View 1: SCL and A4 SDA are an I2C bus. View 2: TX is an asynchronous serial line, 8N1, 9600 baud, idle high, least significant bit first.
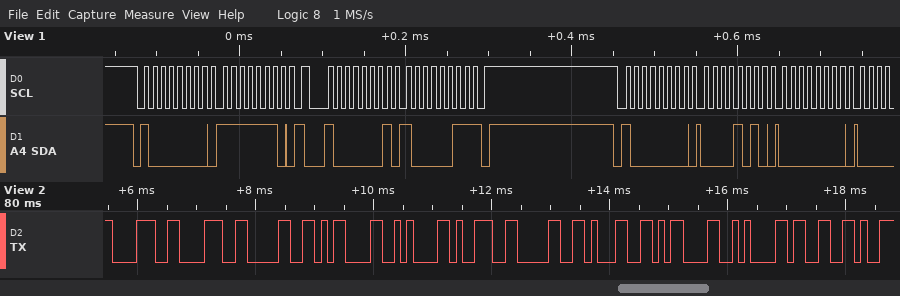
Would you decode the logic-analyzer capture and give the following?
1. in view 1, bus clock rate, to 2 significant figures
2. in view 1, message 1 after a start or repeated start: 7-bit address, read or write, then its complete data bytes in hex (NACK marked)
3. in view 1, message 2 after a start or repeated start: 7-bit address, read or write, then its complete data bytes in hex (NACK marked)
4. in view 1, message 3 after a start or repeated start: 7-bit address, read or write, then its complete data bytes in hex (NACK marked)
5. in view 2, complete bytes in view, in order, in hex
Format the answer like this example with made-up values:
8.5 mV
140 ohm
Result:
100 kHz
0x40 write: FE
0x40 read: 83 NACK
0x40 write: 0A 00
0x38 0x38 0x30 0x0D 0x0A 0x39 0x30 0x31 0x0D 0x0A 0x33
